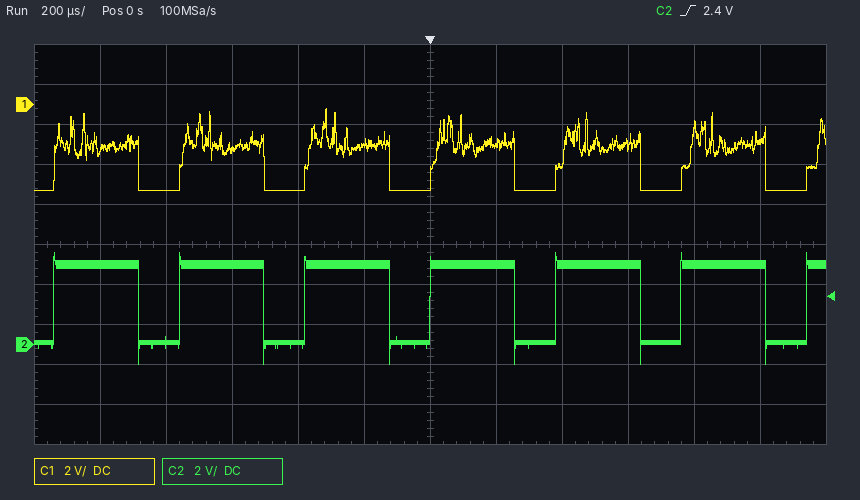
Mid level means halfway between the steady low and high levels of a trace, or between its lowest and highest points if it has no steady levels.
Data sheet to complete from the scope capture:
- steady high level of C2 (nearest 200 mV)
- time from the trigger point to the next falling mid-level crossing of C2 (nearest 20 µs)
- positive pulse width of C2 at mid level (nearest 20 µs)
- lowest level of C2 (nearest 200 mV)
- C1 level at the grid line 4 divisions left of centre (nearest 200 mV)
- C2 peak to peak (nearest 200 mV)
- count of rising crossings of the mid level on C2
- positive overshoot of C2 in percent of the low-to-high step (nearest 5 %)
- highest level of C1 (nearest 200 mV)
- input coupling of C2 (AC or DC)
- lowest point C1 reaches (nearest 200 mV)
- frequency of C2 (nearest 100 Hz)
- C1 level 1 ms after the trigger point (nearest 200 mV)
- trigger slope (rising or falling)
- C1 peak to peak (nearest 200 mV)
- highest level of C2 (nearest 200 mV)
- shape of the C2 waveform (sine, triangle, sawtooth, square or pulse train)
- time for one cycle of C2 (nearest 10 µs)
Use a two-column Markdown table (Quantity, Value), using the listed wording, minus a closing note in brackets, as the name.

| Quantity | Value |
|---|---|
| steady high level of C2 | 4.0 V |
| time from the trigger point to the next falling mid-level crossing of C2 | 260 µs |
| positive pulse width of C2 at mid level | 260 µs |
| lowest level of C2 | -1.0 V |
| C1 level at the grid line 4 divisions left of centre | -4.2 V |
| C2 peak to peak | 5.6 V |
| count of rising crossings of the mid level on C2 | 7 |
| positive overshoot of C2 in percent of the low-to-high step | 15 % |
| highest level of C1 | -200 mV |
| input coupling of C2 | DC |
| lowest point C1 reaches | -4.2 V |
| frequency of C2 | 2.6 kHz |
| C1 level 1 ms after the trigger point | -1.8 V |
| trigger slope | rising |
| C1 peak to peak | 4.0 V |
| highest level of C2 | 4.6 V |
| shape of the C2 waveform | pulse train |
| time for one cycle of C2 | 380 µs |
